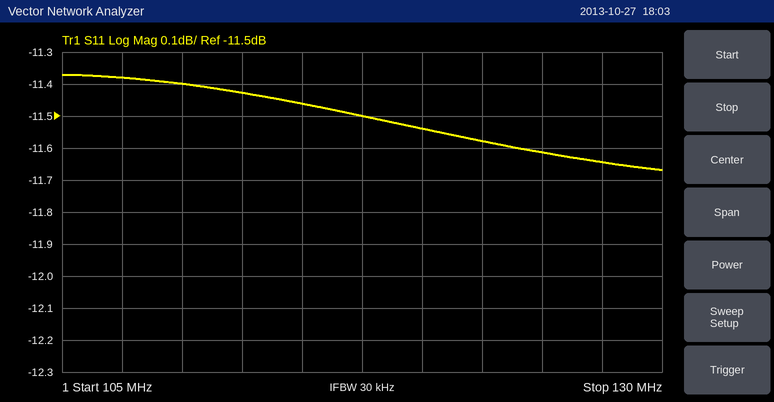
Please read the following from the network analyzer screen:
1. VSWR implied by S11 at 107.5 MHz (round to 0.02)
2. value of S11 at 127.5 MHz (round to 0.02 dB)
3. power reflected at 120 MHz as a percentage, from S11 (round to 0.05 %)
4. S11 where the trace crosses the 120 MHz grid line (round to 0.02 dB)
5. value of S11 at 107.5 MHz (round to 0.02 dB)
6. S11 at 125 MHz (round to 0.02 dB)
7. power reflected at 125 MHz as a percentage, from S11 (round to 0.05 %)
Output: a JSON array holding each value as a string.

["1.74", "-11.64 dB", "7.00 %", "-11.54 dB", "-11.38 dB", "-11.62 dB", "6.90 %"]
